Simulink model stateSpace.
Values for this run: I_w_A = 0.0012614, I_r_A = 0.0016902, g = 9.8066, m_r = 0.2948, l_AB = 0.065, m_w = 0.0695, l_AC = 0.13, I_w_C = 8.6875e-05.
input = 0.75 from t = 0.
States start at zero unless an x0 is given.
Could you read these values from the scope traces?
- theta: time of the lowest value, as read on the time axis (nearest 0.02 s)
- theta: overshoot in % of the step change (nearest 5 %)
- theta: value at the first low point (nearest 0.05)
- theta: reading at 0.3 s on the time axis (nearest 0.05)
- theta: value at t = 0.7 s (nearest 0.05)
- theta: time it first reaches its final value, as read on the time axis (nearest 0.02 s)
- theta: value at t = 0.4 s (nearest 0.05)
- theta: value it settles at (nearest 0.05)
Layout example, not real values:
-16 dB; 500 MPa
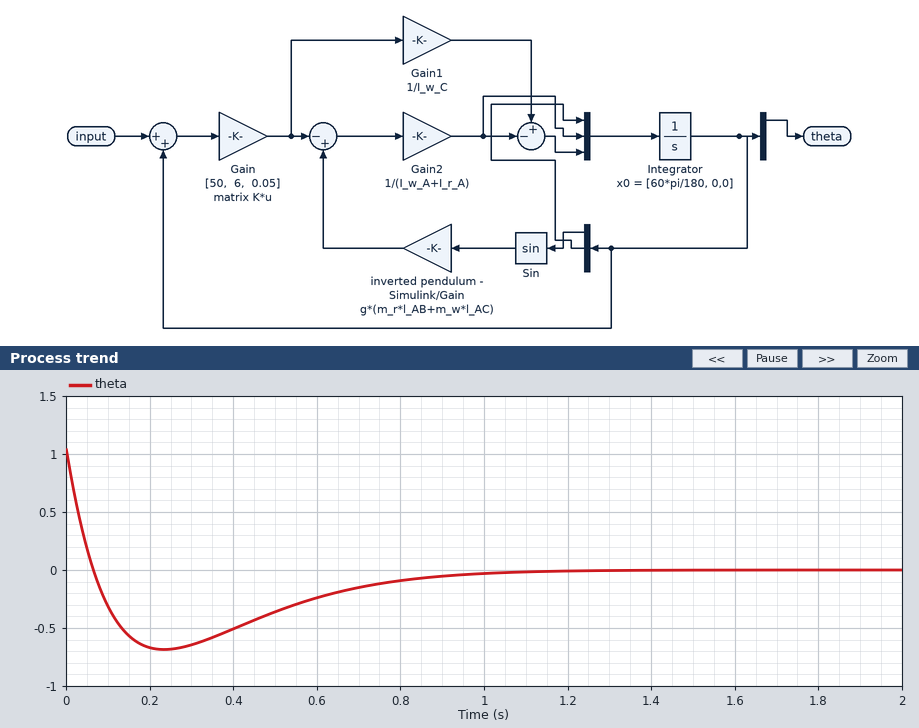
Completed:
0.24 s; 65 %; -0.70; -0.65; -0.15; 0.06 s; -0.50; 0.00
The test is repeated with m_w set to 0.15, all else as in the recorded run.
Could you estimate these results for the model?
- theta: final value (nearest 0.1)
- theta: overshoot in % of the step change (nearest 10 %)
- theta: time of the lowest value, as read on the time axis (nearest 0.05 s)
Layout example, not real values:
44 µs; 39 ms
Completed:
0.0; 60 %; 0.20 s
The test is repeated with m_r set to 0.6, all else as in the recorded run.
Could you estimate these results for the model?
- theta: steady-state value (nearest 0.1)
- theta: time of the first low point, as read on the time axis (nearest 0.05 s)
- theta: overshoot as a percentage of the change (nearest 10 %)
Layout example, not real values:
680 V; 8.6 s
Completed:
0.0; 0.20 s; 60 %
